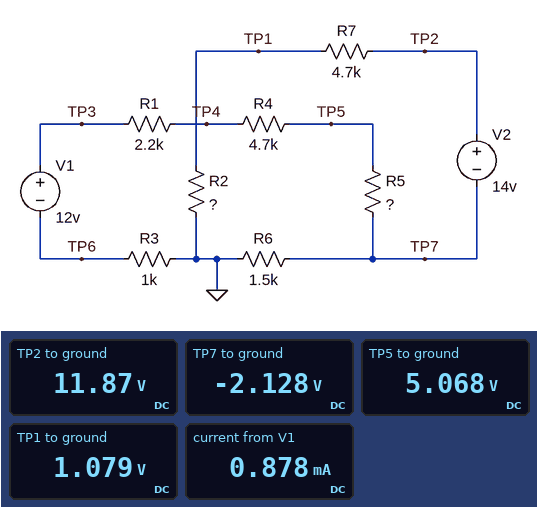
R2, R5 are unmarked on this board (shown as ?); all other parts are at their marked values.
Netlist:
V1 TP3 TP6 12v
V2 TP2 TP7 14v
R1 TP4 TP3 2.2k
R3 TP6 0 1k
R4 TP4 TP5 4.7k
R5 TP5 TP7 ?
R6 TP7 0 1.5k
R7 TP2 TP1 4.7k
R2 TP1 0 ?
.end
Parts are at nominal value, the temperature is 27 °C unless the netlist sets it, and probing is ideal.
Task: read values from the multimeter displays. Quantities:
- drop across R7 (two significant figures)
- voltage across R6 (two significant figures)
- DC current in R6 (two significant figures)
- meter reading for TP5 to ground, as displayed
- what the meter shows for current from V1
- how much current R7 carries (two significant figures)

11 V
2.1 V
1.4 mA
5.068 V
0.878 mA
2.3 mA
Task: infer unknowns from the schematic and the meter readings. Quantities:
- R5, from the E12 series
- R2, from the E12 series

8.2 kΩ
470 Ω
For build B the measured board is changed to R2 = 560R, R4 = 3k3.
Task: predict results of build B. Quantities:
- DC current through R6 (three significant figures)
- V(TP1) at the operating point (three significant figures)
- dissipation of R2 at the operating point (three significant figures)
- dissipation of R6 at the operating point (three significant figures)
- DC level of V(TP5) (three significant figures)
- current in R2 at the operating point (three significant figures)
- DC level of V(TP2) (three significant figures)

1.33 mA
1.28 V
2.92 mW
2.65 mW
5.81 V
2.28 mA
12.0 V
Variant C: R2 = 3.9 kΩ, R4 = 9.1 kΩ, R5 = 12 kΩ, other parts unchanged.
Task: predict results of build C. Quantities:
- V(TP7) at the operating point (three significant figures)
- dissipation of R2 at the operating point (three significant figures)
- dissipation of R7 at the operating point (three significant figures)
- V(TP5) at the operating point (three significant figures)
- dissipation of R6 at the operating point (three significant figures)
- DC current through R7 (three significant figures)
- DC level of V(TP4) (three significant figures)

-1.38 V
8.40 mW
10.1 mW
5.23 V
1.26 mW
1.47 mA
10.2 V
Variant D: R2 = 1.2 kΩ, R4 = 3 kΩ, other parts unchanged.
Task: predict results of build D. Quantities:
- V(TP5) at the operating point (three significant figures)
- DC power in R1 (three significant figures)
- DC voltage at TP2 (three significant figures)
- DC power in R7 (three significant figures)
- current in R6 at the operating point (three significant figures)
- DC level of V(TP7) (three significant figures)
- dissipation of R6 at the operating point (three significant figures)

6.10 V
1.99 mW
12.3 V
20.4 mW
1.13 mA
-1.70 V
1.93 mW
